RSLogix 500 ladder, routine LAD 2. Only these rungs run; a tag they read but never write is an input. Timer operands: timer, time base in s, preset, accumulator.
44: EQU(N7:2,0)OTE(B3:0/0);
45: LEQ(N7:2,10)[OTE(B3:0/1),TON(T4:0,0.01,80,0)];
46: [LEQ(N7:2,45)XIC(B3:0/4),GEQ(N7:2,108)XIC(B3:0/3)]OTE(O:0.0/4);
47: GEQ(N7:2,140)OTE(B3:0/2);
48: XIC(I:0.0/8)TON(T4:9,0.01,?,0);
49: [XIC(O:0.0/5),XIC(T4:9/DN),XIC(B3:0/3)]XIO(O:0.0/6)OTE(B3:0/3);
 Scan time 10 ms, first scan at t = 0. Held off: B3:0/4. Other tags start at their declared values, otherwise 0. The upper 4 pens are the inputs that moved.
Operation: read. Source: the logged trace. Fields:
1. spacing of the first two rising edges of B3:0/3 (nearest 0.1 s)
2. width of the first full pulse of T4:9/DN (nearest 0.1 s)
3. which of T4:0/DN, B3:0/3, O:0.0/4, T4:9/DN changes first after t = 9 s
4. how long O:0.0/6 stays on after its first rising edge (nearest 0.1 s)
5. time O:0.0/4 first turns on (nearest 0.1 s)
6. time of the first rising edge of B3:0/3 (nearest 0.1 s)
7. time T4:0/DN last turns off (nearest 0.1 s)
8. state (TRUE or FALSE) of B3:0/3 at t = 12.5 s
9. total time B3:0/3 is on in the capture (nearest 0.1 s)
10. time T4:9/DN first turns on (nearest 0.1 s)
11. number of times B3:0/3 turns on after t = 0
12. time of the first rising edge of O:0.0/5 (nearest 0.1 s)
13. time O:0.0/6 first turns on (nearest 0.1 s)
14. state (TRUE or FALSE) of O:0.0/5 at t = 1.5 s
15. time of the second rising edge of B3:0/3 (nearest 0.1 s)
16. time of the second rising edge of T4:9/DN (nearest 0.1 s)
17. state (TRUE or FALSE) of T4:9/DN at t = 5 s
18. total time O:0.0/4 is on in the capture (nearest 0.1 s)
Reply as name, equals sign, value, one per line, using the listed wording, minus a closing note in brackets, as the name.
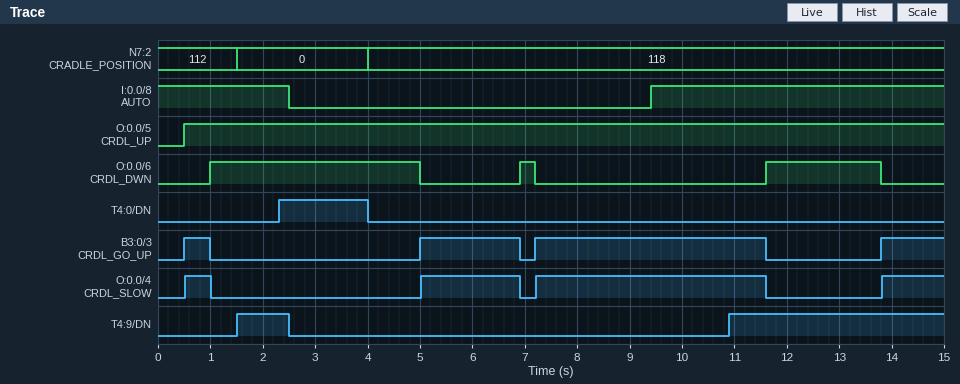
spacing of the first two rising edges of B3:0/3 = 4.5 s
width of the first full pulse of T4:9/DN = 1.0 s
which of T4:0/DN, B3:0/3, O:0.0/4, T4:9/DN changes first after t = 9 s = T4:9/DN
how long O:0.0/6 stays on after its first rising edge = 4.0 s
time O:0.0/4 first turns on = 0.5 s
time of the first rising edge of B3:0/3 = 0.5 s
time T4:0/DN last turns off = 4.0 s
state (TRUE or FALSE) of B3:0/3 at t = 12.5 s = FALSE
total time B3:0/3 is on in the capture = 8.0 s
time T4:9/DN first turns on = 1.5 s
number of times B3:0/3 turns on after t = 0 = 4
time of the first rising edge of O:0.0/5 = 0.5 s
time O:0.0/6 first turns on = 1.0 s
state (TRUE or FALSE) of O:0.0/5 at t = 1.5 s = TRUE
time of the second rising edge of B3:0/3 = 5.0 s
time of the second rising edge of T4:9/DN = 10.9 s
state (TRUE or FALSE) of T4:9/DN at t = 5 s = FALSE
total time O:0.0/4 is on in the capture = 8.0 s
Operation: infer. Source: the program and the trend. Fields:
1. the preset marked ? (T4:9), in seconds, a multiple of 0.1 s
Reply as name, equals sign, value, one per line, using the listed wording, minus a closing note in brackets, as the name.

the preset marked ? (T4:9), in seconds, a multiple of 0.1 s = 1.5 s
